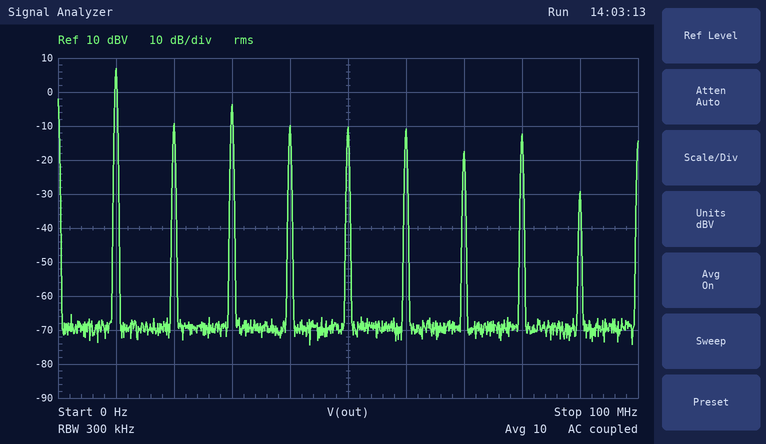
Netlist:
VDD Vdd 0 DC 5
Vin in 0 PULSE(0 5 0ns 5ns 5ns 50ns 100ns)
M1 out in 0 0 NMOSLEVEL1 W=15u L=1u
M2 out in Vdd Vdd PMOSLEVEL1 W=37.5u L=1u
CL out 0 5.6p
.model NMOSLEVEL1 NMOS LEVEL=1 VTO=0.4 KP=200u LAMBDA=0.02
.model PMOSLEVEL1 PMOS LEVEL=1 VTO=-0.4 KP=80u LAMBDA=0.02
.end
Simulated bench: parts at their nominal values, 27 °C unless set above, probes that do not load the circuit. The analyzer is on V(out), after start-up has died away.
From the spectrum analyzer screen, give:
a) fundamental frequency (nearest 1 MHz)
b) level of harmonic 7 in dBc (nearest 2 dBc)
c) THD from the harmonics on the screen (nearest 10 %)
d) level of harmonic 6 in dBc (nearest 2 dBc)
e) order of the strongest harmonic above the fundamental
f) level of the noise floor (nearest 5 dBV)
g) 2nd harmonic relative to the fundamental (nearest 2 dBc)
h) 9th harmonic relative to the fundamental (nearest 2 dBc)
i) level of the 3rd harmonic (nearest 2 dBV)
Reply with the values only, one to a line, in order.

10 MHz
-24 dBc
40 %
-18 dBc
3
-70 dBV
-16 dBc
-36 dBc
-4 dBV
